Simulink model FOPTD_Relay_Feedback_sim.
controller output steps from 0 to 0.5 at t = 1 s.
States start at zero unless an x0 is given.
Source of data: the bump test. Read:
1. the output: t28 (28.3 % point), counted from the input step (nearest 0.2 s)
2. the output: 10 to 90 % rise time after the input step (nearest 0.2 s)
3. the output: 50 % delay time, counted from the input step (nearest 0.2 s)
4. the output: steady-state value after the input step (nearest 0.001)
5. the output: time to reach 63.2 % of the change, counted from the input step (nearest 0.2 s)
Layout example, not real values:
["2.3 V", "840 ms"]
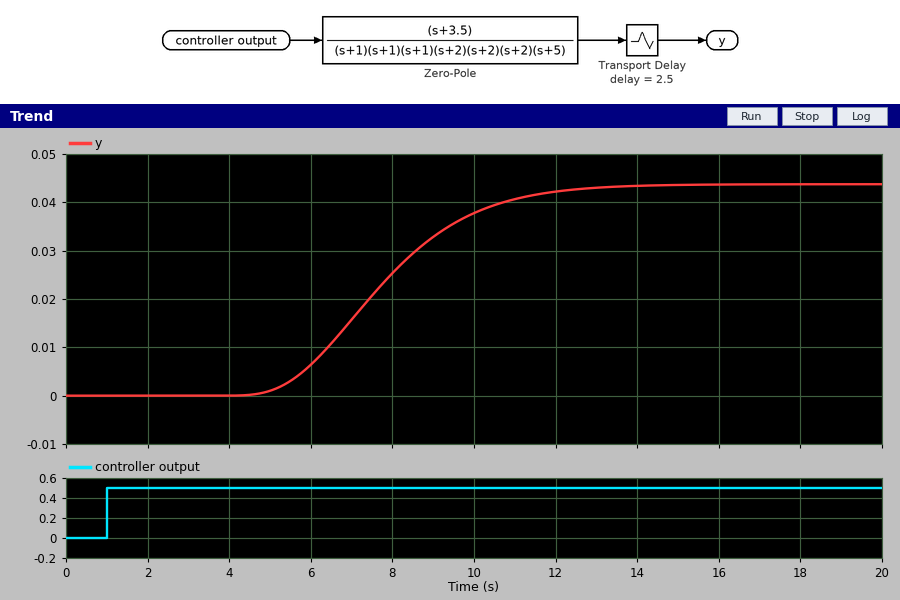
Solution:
["5.6 s", "4.8 s", "6.6 s", "0.044", "7.2 s"]
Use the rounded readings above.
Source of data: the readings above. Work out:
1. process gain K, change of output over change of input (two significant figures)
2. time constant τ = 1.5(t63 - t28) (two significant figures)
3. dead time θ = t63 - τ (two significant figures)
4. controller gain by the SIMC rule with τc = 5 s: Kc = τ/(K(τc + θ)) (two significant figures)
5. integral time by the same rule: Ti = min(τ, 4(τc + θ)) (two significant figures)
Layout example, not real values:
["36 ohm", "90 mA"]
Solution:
["0.088", "2.4 s", "4.8 s", "2.8", "2.4 s"]
